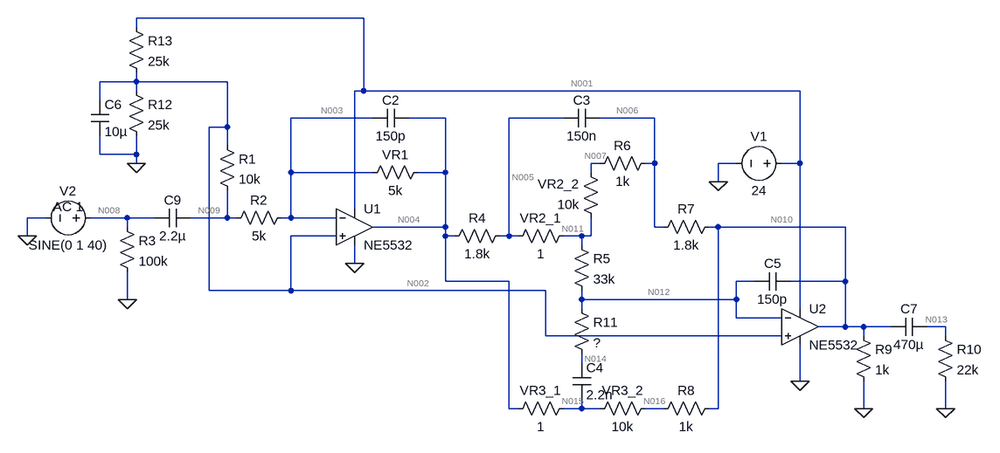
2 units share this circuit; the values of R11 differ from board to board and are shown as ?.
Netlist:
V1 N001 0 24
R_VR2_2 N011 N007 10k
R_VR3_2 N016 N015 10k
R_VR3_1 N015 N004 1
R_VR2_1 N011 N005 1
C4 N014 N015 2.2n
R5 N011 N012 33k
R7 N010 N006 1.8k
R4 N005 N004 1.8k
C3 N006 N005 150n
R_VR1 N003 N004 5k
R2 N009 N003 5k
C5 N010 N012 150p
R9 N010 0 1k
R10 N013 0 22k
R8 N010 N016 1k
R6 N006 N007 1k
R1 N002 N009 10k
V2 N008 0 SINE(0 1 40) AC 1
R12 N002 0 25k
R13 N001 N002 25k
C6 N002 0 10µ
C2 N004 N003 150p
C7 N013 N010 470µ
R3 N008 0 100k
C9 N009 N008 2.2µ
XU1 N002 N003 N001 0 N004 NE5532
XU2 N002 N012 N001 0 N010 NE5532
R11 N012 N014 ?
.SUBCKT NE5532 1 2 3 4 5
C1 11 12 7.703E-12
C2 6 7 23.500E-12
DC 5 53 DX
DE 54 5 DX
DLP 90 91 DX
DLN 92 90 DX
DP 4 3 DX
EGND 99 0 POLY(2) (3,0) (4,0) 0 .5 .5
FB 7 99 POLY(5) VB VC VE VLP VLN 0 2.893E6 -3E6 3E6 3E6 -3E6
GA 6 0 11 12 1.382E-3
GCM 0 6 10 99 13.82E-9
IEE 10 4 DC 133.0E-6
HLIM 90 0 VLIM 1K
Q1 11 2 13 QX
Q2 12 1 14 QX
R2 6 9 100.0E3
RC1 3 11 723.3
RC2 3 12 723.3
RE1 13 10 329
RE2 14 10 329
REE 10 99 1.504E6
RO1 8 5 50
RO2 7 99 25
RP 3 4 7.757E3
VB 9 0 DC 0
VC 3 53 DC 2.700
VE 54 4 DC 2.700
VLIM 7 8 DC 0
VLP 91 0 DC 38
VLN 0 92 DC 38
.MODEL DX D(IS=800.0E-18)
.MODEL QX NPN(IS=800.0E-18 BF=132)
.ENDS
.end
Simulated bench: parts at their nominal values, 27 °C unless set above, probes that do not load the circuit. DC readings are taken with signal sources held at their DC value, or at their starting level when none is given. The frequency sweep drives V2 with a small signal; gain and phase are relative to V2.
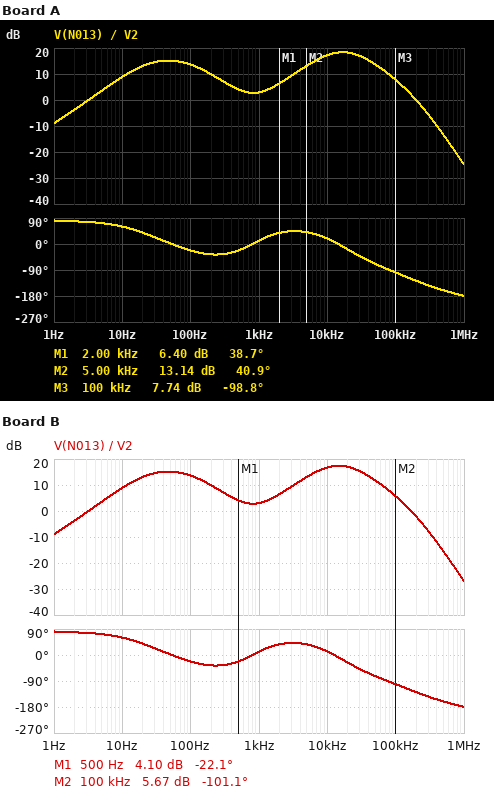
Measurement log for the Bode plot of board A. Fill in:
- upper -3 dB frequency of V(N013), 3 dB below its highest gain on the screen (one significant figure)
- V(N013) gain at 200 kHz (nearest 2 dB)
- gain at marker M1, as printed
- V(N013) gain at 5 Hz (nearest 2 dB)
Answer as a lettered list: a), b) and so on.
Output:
a) 40 kHz
b) 0 dB
c) 6.40 dB
d) 4 dB
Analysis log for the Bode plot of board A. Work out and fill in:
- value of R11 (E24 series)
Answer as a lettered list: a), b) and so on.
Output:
a) 3.9 kΩ
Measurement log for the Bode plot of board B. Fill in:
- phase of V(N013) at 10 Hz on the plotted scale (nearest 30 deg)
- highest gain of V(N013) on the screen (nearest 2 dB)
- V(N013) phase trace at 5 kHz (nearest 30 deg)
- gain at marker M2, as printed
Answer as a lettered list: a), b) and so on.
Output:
a) 60 deg
b) 18 dB
c) 30 deg
d) 5.67 dB
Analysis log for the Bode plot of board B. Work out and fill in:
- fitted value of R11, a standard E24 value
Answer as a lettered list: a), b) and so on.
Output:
a) 5.1 kΩ
